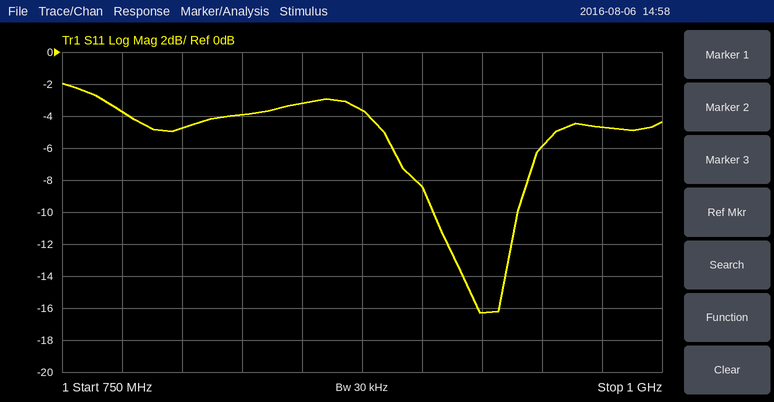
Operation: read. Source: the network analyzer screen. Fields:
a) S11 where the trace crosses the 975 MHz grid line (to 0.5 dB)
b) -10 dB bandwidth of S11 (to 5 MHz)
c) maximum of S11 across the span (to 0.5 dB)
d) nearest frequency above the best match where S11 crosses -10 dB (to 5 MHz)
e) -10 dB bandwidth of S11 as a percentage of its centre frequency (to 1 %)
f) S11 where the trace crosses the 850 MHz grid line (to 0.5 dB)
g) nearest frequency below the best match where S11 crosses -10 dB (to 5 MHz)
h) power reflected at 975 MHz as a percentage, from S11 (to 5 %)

-4.5 dB
35 MHz
-2.0 dB
940 MHz
4 %
-3.0 dB
905 MHz
35 %
